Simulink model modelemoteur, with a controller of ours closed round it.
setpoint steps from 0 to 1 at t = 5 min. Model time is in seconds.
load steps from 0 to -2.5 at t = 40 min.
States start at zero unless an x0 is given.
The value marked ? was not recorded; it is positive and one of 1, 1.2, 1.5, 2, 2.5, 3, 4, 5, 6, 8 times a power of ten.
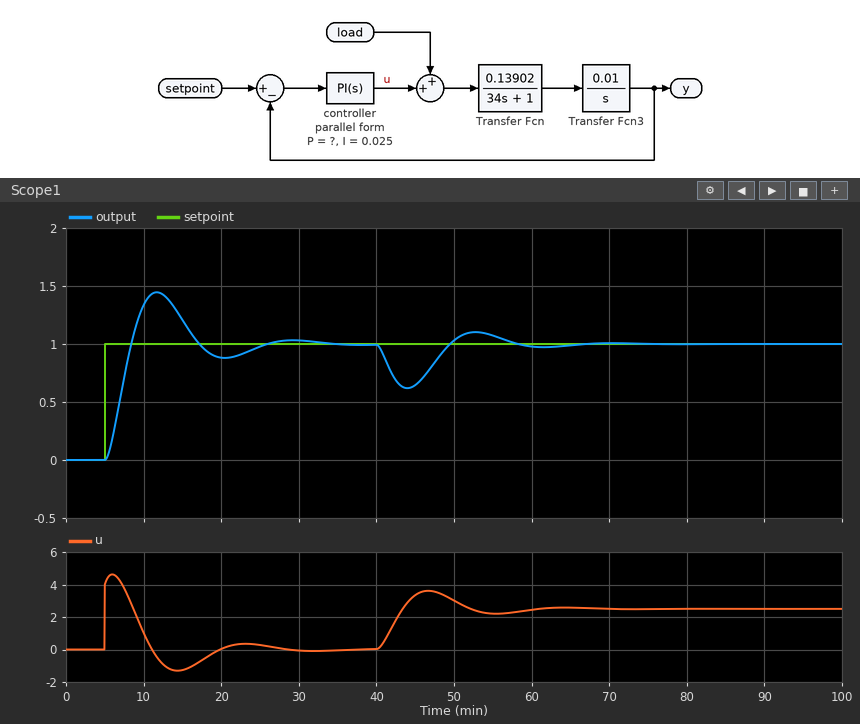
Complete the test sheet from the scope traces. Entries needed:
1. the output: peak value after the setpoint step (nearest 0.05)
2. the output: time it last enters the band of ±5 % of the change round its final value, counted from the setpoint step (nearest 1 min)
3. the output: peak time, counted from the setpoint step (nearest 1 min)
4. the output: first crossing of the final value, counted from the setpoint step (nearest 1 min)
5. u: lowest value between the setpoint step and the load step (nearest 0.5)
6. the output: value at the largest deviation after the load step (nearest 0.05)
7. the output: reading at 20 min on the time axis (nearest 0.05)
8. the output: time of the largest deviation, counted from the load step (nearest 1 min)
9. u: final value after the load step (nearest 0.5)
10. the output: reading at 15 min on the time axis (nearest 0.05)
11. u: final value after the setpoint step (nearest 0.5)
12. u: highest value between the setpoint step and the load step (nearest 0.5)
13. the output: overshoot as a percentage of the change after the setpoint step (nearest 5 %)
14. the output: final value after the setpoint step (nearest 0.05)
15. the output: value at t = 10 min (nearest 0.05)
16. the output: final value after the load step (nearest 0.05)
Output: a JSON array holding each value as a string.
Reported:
["1.45", "19 min", "7 min", "3 min", "-1.5", "0.60", "0.90", "4 min", "2.5", "1.20", "0.0", "4.5", "45 %", "1.00", "1.35", "1.00"]
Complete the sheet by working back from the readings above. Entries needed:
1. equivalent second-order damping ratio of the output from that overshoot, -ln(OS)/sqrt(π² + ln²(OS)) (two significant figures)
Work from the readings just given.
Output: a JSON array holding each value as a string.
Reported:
["0.25"]
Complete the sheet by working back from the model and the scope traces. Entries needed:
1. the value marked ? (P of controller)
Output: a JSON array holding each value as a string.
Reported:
["4"]
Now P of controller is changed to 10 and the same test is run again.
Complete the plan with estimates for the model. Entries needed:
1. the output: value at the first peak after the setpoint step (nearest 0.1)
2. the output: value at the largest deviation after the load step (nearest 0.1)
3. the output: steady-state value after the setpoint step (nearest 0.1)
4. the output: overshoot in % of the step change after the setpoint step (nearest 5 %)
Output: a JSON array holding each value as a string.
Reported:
["1.2", "0.8", "1.0", "20 %"]
